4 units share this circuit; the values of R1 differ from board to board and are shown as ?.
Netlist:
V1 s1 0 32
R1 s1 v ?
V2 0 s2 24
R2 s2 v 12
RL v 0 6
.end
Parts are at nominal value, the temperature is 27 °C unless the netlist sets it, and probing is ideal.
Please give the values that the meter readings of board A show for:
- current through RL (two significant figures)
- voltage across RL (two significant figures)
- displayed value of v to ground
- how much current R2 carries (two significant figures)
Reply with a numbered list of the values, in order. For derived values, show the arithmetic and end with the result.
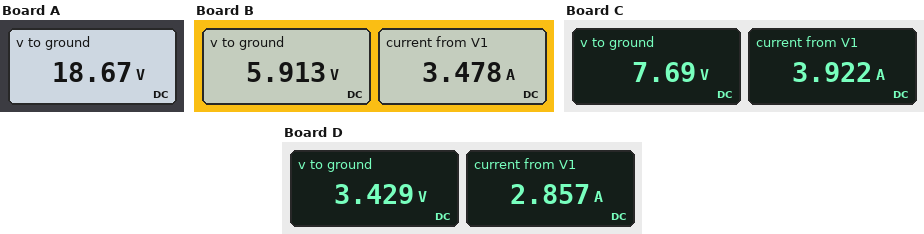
1. (18.67 V) / 6 Ω = 3.1 A
2. 18.67 V = 19 V
3. 18.67 V
4. (18.67 V - (-24 V)) / 12 Ω = 3.6 A
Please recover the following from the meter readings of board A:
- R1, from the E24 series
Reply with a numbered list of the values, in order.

1. 2 Ω
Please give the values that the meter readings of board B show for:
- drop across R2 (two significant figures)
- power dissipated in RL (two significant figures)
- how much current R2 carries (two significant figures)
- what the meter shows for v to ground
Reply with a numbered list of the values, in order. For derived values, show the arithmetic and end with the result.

1. 5.913 V - (-24 V) = 30 V
2. (5.913 V)^2 / 6 Ω = 5.8 W
3. (5.913 V - (-24 V)) / 12 Ω = 2.5 A
4. 5.913 V
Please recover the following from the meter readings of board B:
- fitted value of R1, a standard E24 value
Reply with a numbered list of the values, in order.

1. 7.5 Ω
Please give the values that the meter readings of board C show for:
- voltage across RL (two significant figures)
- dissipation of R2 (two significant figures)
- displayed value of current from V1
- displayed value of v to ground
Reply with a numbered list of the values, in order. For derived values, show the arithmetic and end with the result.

1. 7.69 V = 7.7 V
2. (7.69 V - (-24 V))^2 / 12 Ω = 84 W
3. 3.922 A
4. 7.69 V
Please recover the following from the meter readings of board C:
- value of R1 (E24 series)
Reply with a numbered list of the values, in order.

1. 6.2 Ω
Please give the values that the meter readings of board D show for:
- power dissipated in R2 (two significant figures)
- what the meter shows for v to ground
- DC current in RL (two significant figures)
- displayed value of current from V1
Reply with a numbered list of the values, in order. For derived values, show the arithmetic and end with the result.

1. (3.429 V - (-24 V))^2 / 12 Ω = 63 W
2. 3.429 V
3. (3.429 V) / 6 Ω = 570 mA
4. 2.857 A
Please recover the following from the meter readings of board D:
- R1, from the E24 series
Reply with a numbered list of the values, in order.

1. 10 Ω
